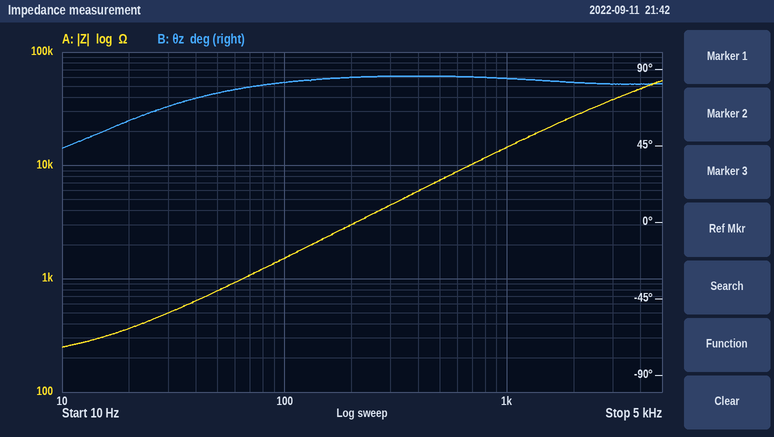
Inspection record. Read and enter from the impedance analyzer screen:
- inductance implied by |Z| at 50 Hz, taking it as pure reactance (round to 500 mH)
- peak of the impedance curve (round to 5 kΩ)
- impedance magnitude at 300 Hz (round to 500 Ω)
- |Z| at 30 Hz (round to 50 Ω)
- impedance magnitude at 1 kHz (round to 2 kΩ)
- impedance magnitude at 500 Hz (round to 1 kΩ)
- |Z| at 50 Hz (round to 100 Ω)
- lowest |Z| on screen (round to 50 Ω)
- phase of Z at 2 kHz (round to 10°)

2.5 H
55 kΩ
4.5 kΩ
500 Ω
14 kΩ
7 kΩ
800 Ω
250 Ω
80°
